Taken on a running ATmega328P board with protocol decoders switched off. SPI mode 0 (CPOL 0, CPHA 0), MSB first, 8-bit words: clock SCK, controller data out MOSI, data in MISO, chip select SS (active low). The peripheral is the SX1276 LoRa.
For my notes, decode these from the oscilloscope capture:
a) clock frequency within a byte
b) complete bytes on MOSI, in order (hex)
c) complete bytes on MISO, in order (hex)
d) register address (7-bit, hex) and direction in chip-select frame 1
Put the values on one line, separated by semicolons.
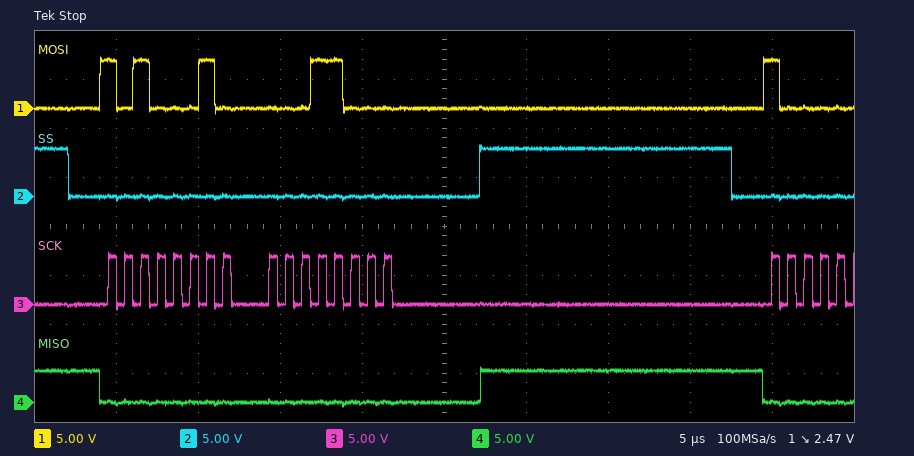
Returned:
1 MHz; 0xA2 0x18; 0x00 0x00; 0x22 write
